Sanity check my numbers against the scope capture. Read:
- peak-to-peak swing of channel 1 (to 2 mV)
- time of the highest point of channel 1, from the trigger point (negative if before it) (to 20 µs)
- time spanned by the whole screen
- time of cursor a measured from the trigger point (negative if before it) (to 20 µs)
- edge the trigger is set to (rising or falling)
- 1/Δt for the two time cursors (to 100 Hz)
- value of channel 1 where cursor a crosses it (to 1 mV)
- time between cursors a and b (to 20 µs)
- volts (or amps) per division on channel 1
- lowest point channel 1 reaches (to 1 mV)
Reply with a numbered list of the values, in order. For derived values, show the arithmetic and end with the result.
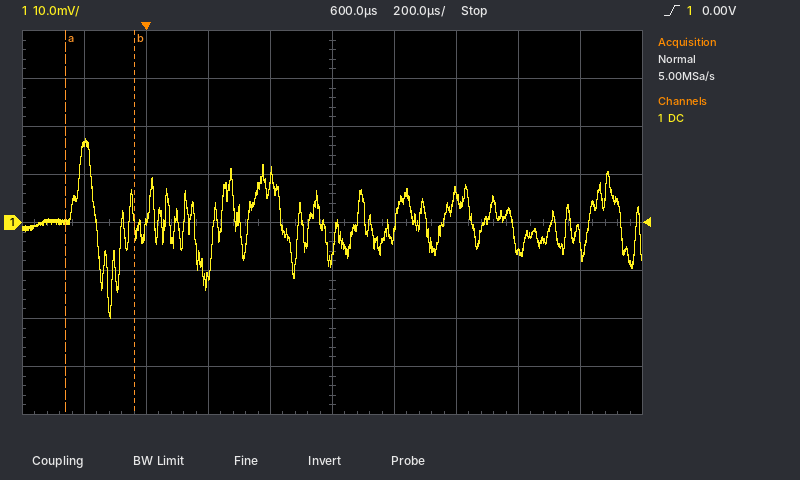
1. 38 mV
2. -200 µs
3. 2 ms
4. -260 µs
5. rising
6. 1 / 220 µs ≈ 4.5 kHz
7. 0 mV
8. 220 µs
9. 10 mV
10. -20 mV
